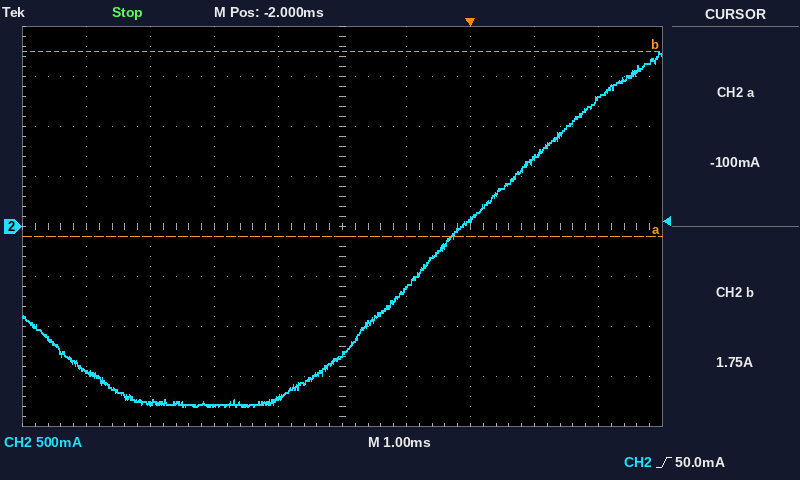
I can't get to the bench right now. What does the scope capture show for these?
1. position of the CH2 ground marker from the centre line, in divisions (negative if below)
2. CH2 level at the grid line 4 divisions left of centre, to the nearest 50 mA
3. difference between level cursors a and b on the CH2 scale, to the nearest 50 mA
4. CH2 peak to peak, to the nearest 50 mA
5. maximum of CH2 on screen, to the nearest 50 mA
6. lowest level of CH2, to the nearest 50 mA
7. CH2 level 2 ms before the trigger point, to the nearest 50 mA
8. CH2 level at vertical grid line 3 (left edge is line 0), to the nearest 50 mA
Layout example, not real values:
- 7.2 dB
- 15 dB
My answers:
- 0.0 div
- -1.45 A
- 1.85 A
- 3.55 A
- 1.75 A
- -1.80 A
- -1.30 A
- -1.80 A
